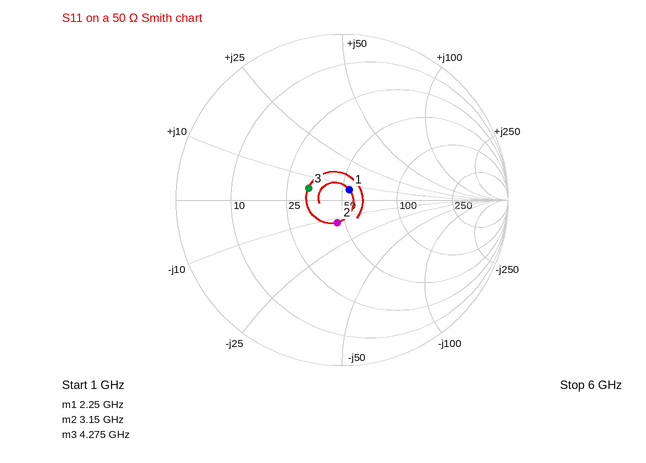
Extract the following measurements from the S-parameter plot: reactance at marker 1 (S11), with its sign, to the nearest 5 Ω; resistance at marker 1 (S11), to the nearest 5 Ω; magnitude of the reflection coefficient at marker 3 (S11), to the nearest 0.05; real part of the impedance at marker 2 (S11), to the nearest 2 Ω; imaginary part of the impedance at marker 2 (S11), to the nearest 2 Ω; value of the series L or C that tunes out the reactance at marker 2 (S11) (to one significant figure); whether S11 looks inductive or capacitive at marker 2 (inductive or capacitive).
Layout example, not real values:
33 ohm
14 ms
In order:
+5 Ω
55 Ω
0.20
46 Ω
-12 Ω
600 pH
capacitive
